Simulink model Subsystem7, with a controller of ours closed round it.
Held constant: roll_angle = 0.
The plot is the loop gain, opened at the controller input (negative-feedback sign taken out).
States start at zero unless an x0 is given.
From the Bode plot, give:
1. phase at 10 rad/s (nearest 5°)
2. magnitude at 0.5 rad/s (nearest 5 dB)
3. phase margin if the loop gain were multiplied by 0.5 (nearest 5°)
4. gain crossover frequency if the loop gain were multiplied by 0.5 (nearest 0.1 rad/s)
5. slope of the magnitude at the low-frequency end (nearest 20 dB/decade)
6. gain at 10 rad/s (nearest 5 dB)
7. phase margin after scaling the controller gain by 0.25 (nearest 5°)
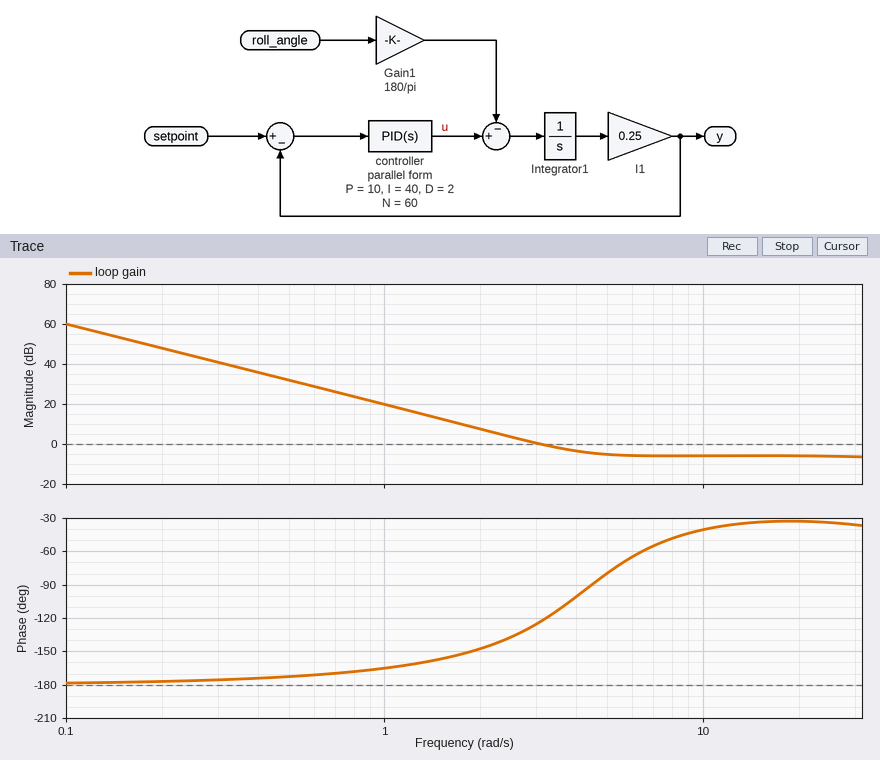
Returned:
-40°
30 dB
35°
2.2 rad/s
-40 dB/decade
-5 dB
25°
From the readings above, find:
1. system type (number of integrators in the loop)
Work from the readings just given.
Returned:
2
